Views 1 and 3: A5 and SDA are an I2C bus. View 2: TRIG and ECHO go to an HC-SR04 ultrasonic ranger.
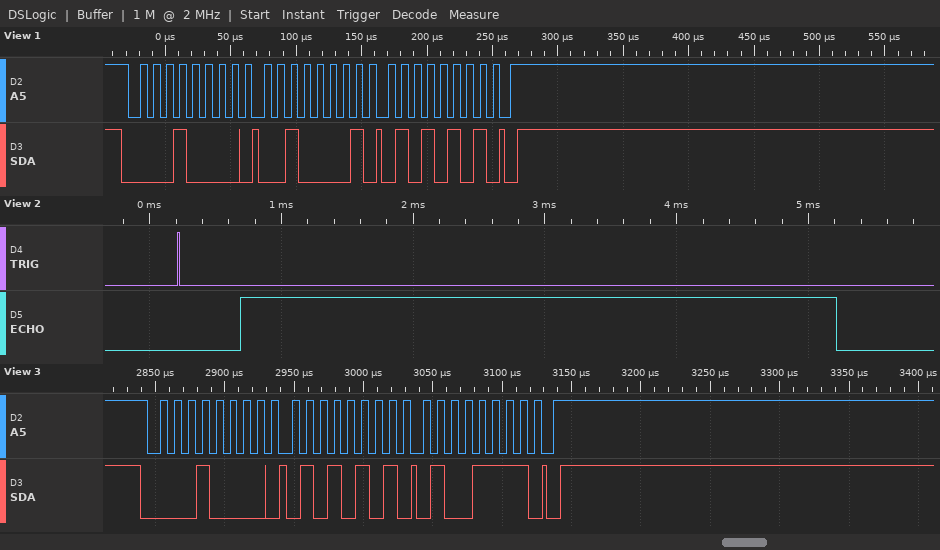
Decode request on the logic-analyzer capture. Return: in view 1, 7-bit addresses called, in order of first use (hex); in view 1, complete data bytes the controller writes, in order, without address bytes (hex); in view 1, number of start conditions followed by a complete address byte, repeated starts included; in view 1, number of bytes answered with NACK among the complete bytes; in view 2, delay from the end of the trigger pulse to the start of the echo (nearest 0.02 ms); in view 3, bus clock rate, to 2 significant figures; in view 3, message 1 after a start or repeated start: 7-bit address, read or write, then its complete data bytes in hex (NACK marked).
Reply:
0x08
21 55
1
0
0.46 ms
100 kHz
0x08 write: 55 4F
